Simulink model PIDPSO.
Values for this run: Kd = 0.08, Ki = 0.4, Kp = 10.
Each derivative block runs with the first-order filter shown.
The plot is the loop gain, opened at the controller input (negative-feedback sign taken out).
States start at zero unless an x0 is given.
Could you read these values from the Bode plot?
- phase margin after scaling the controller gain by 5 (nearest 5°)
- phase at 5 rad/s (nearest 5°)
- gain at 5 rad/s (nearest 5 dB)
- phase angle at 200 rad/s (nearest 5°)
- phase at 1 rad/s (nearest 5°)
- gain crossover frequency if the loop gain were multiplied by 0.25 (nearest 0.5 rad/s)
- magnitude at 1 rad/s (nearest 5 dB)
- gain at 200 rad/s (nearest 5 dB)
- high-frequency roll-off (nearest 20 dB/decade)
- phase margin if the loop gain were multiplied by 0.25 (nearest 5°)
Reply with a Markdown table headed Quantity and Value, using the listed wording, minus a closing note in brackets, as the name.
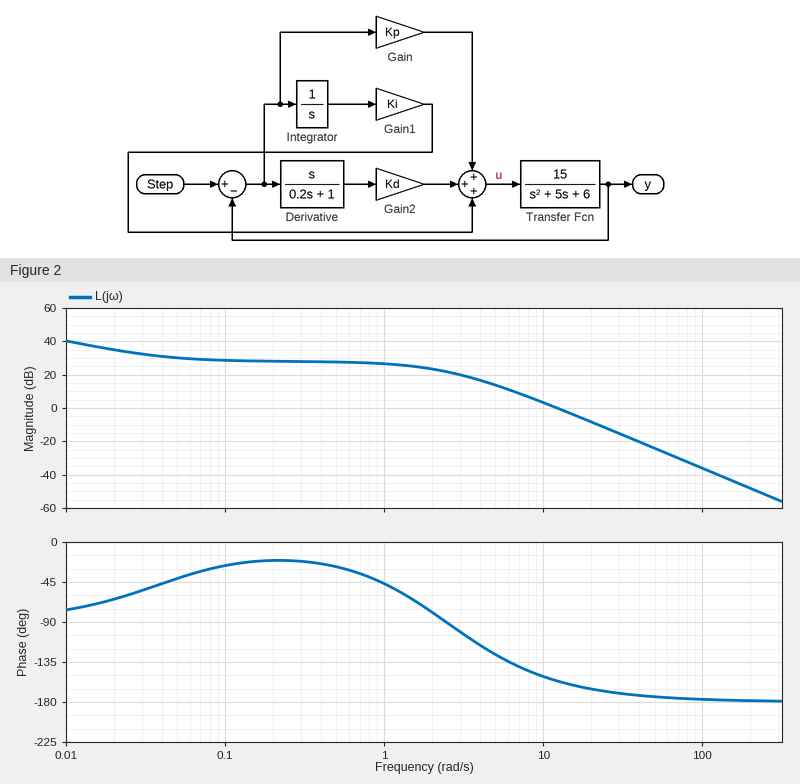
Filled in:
| Quantity | Value |
|---|---|
| phase margin after scaling the controller gain by 5 | 10° |
| phase at 5 rad/s | -125° |
| gain at 5 rad/s | 15 dB |
| phase angle at 200 rad/s | -180° |
| phase at 1 rad/s | -45° |
| gain crossover frequency if the loop gain were multiplied by 0.25 | 5.5 rad/s |
| magnitude at 1 rad/s | 25 dB |
| gain at 200 rad/s | -50 dB |
| high-frequency roll-off | -40 dB/decade |
| phase margin if the loop gain were multiplied by 0.25 | 50° |
